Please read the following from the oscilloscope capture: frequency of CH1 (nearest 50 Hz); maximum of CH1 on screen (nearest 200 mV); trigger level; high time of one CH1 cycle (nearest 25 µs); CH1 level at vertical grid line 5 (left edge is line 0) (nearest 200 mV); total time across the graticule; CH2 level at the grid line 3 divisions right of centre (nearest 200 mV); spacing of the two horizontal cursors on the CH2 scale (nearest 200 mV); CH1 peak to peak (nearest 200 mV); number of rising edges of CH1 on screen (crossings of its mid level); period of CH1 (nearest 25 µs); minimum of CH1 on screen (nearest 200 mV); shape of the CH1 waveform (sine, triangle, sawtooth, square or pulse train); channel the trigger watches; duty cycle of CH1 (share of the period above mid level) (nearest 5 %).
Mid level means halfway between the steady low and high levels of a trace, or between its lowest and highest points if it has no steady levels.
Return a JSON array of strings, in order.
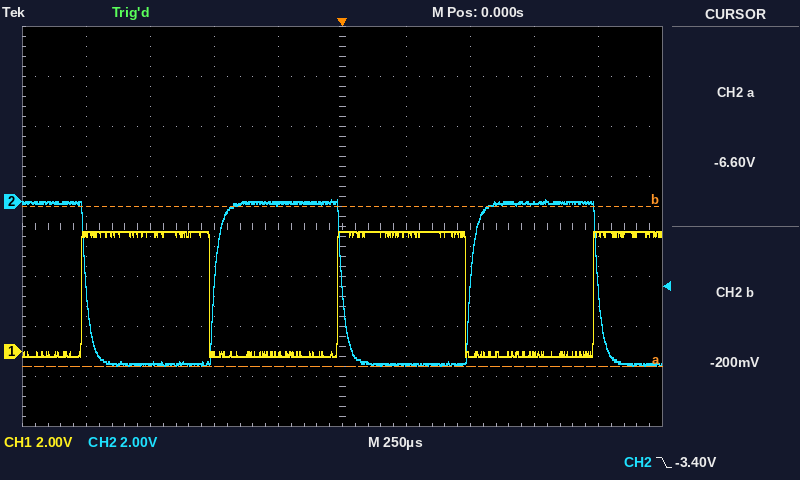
["1.00 kHz", "4.8 V", "-3.40 V", "500 µs", "4.8 V", "2.5 ms", "0.0 V", "6.4 V", "5.0 V", "3", "1.000 ms", "-200 mV", "square", "CH2", "50 %"]
